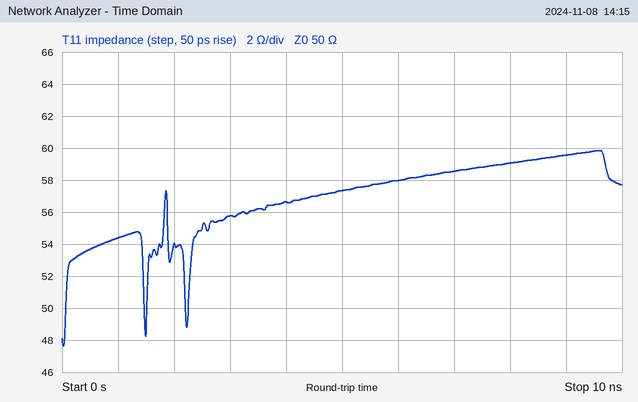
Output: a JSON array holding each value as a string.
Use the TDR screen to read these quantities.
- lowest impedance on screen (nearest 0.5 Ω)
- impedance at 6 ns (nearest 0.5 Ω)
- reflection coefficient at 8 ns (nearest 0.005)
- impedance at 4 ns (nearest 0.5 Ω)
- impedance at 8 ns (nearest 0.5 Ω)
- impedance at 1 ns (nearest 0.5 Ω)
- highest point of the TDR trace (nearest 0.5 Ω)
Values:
["47.5 Ω", "58.0 Ω", "+0.085", "56.5 Ω", "59.0 Ω", "54.5 Ω", "60.0 Ω"]
